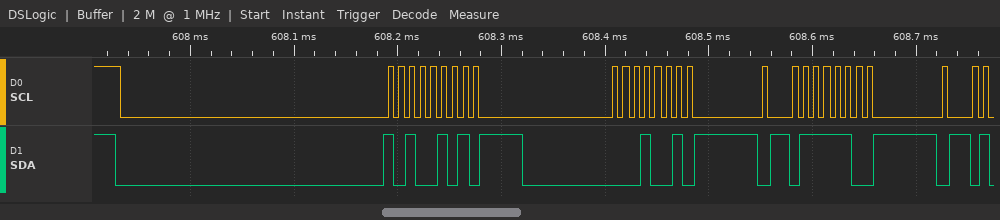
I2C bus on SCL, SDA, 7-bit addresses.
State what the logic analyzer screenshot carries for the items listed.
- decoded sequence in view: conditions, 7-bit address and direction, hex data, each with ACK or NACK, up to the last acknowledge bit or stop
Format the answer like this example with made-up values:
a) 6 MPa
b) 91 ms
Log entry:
a) start, address 52 read ACK, 12 ACK, 7C ACK
